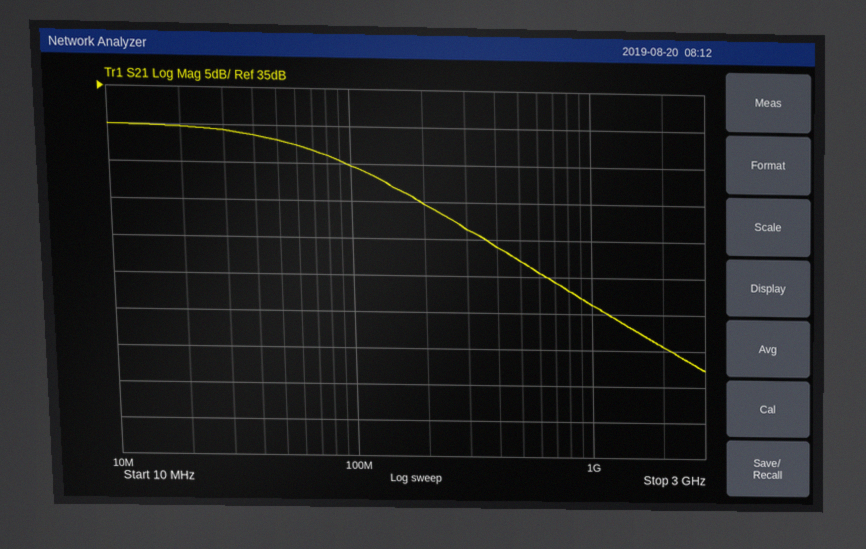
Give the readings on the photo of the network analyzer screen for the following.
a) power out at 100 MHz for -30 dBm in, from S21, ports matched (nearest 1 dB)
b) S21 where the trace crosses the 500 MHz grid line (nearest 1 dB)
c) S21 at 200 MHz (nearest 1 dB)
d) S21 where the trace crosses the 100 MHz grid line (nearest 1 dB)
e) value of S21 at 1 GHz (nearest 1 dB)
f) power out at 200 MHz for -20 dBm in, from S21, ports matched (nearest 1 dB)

-5 dBm
12 dB
20 dB
25 dB
6 dB
0 dBm
